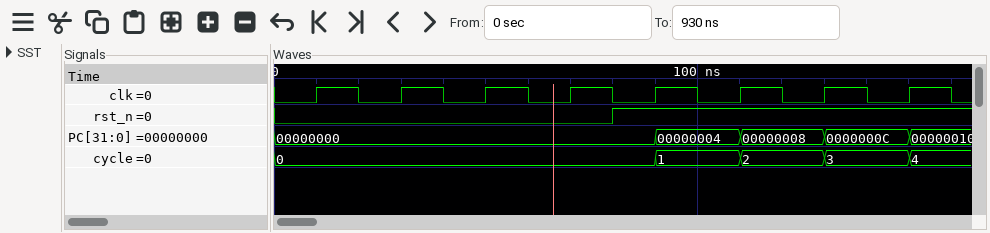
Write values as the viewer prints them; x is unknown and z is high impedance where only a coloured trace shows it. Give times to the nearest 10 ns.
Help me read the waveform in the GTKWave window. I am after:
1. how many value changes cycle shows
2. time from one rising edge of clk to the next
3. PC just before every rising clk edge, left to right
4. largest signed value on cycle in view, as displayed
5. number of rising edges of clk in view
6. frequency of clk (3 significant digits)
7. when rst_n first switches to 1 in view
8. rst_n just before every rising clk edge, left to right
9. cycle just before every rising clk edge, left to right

4
20 ns
00000000, 00000000, 00000000, 00000000, 00000000, 00000004, 00000008, 0000000C
4
8
50.0 MHz
80 ns
0 0 0 0 1 1 1 1
0, 0, 0, 0, 0, 1, 2, 3
